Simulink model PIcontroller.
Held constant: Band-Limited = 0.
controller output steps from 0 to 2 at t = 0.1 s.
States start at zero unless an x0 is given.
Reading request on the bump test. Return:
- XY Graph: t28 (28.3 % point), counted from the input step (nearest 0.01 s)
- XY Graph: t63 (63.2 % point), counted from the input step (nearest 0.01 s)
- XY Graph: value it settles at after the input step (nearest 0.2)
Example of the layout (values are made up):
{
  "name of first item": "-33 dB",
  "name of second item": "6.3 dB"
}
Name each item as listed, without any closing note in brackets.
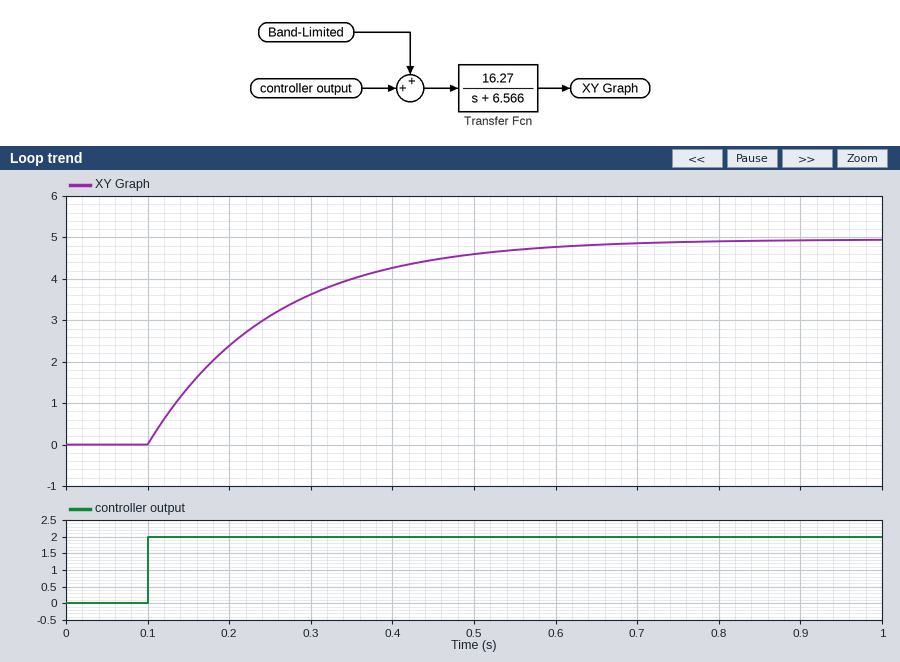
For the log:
{
  "XY Graph: t28 (28.3 % point), counted from the input step": "0.05 s",
  "XY Graph: t63 (63.2 % point), counted from the input step": "0.15 s",
  "XY Graph: value it settles at after the input step": "5.0"
}
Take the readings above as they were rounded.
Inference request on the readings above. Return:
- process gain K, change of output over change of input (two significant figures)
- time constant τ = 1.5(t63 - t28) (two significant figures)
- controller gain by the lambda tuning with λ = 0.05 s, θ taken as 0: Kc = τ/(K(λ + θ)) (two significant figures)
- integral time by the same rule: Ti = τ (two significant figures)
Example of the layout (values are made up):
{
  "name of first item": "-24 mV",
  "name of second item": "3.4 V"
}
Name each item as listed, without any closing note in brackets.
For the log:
{
  "process gain K, change of output over change of input": "2.5",
  "time constant τ = 1.5(t63 - t28)": "0.15 s",
  "controller gain by the lambda tuning with λ = 0.05 s, θ taken as 0: Kc = τ/(K(λ + θ))": "1.2",
  "integral time by the same rule: Ti = τ": "0.15 s"
}
